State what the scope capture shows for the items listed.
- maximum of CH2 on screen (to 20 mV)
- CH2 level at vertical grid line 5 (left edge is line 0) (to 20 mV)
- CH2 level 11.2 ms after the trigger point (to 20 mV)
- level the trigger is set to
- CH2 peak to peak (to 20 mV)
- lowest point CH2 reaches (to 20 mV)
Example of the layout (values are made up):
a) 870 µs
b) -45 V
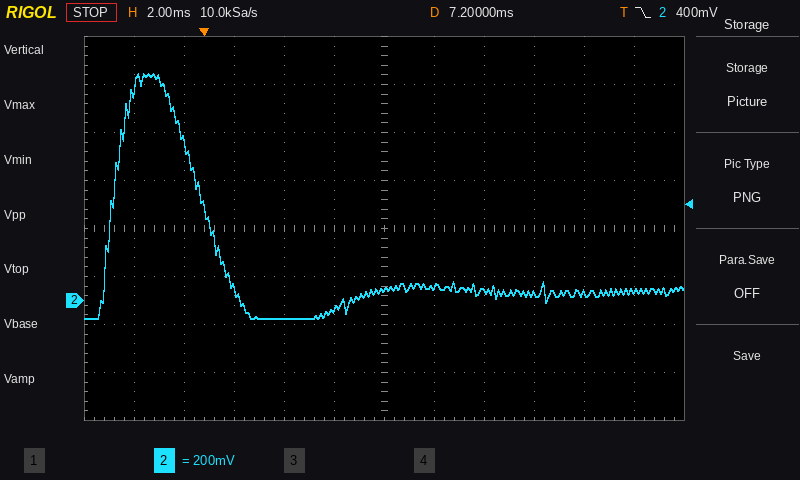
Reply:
a) 940 mV
b) -40 mV
c) 40 mV
d) 400 mV
e) 1.02 V
f) -80 mV
